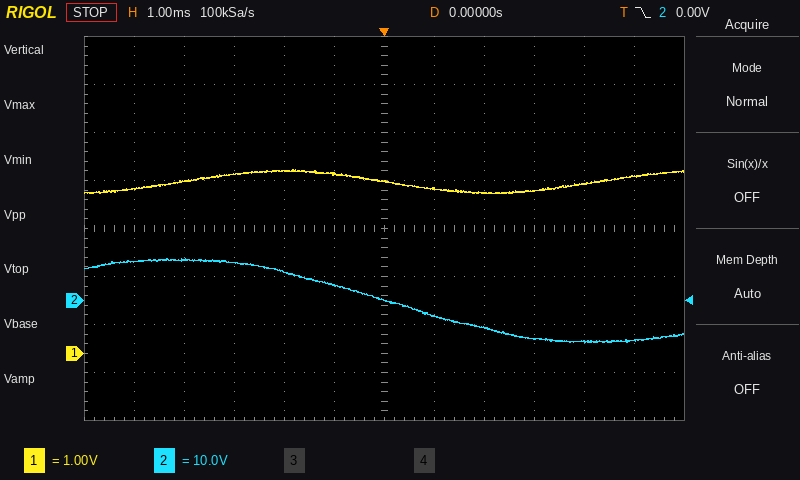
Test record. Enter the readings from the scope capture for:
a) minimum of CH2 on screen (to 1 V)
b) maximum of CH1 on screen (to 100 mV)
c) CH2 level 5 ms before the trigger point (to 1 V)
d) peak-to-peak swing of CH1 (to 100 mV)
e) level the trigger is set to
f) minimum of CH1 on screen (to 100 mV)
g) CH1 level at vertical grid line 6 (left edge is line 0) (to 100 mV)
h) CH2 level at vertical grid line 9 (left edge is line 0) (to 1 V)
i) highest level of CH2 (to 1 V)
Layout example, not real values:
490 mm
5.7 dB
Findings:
-9 V
3.8 V
8 V
500 mV
0.00 V
3.3 V
3.6 V
-8 V
9 V
